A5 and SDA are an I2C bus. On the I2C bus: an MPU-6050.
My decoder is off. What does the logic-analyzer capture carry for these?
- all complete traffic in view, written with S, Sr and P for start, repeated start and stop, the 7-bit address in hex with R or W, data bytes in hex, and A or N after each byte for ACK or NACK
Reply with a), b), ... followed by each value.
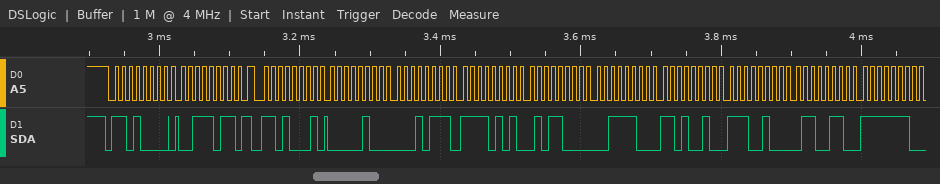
a) S 68W A 3B A Sr 68R A 04 A 17 A F5 A 58 A 3C A D2 A E4 A 66 A FE A
